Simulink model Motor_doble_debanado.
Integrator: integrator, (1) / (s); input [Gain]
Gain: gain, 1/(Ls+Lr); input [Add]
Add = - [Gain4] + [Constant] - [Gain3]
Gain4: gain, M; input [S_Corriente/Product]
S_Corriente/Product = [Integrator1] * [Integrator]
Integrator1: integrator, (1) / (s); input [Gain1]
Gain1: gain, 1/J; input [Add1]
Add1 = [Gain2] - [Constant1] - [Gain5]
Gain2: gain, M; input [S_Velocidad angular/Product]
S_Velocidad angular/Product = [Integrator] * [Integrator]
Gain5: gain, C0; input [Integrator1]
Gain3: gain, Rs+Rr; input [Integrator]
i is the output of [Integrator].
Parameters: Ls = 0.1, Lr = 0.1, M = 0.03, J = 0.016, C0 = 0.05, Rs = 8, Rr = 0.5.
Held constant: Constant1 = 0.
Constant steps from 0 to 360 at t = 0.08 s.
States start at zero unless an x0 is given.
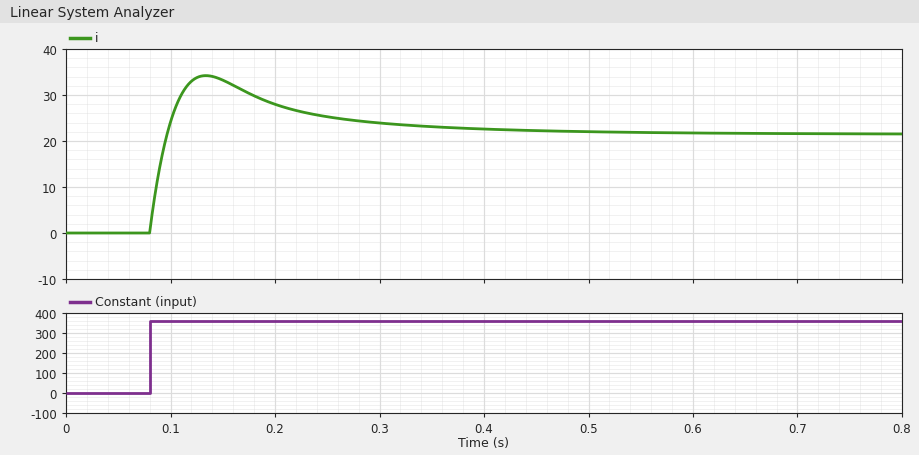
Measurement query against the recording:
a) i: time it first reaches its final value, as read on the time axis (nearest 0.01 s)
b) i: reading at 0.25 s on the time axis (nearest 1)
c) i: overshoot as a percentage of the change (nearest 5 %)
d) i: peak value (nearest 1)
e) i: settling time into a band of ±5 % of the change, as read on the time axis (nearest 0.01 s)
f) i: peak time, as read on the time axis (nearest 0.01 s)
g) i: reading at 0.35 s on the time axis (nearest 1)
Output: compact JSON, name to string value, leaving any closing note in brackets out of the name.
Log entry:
{"i: time it first reaches its final value, as read on the time axis": "0.10 s", "i: reading at 0.25 s on the time axis": "25", "i: overshoot as a percentage of the change": "60 %", "i: peak value": "34", "i: settling time into a band of ±5 % of the change, as read on the time axis": "0.41 s", "i: peak time, as read on the time axis": "0.13 s", "i: reading at 0.35 s on the time axis": "23"}
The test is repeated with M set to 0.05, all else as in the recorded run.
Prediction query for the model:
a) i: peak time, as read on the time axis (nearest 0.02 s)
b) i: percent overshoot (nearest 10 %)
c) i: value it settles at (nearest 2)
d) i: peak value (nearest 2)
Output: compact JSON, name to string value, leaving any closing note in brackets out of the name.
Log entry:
{"i: peak time, as read on the time axis": "0.12 s", "i: percent overshoot": "90 %", "i: value it settles at": "16", "i: peak value": "30"}
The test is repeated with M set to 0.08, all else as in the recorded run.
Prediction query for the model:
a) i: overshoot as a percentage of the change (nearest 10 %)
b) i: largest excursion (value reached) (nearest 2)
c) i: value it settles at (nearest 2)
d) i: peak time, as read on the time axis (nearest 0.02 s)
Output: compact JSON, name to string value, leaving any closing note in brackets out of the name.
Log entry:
{"i: overshoot as a percentage of the change": "110 %", "i: largest excursion (value reached)": "26", "i: value it settles at": "12", "i: peak time, as read on the time axis": "0.12 s"}
